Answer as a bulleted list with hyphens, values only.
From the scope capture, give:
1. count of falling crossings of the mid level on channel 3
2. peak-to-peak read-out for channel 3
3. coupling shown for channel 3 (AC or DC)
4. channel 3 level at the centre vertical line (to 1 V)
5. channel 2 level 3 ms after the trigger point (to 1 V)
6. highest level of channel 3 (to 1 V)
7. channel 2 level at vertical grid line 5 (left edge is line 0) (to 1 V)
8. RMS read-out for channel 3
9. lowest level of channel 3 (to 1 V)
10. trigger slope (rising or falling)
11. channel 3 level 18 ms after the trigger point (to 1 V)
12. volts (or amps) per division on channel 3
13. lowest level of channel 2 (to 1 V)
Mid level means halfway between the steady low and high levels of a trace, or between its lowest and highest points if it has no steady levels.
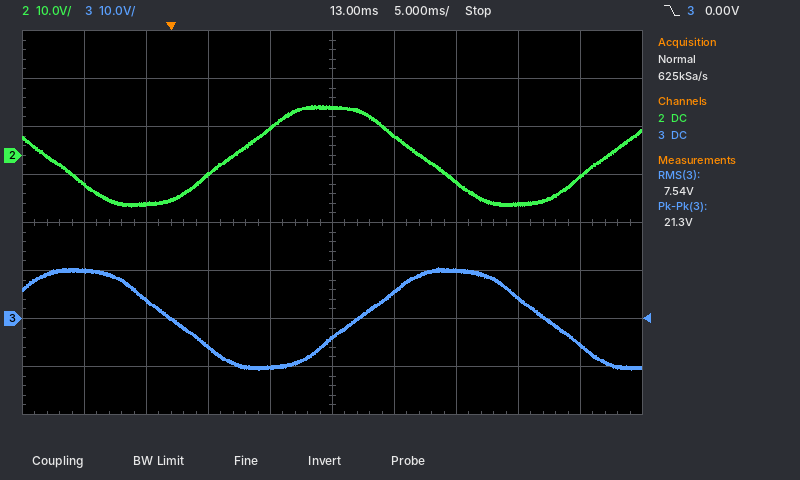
- 2
- 21.3 V
- DC
- -4 V
- -4 V
- 11 V
- 10 V
- 7.54 V
- -11 V
- falling
- 6 V
- 10 V
- -11 V
